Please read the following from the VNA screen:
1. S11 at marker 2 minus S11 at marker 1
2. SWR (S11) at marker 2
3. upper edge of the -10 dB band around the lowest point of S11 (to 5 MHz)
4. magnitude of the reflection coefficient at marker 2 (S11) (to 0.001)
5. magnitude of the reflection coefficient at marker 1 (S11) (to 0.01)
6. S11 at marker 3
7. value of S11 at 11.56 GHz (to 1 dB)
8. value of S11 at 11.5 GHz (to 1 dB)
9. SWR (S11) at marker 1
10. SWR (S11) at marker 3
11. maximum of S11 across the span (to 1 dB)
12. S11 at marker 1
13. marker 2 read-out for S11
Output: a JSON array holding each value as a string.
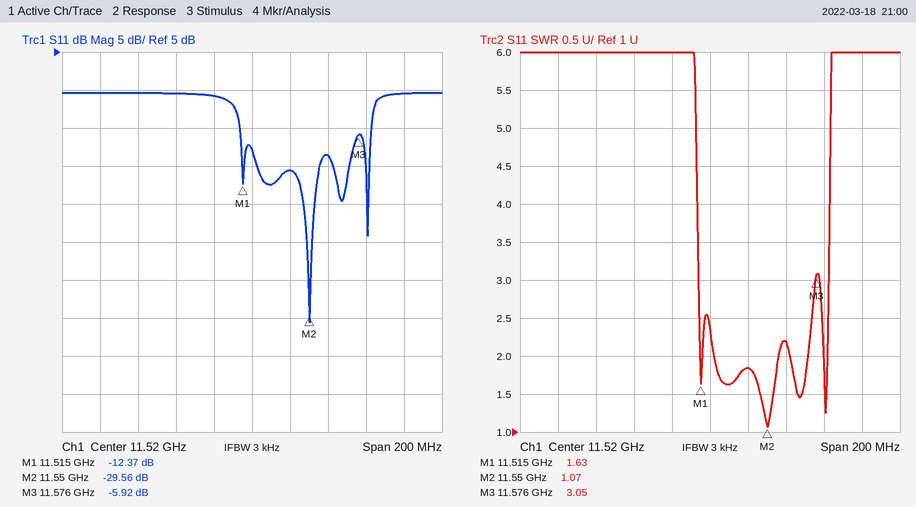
["-17.19 dB", "1.07", "11.555 GHz", "0.033", "0.24", "-5.92 dB", "-9 dB", "-1 dB", "1.63", "3.05", "0 dB", "-12.37 dB", "-29.56 dB"]
